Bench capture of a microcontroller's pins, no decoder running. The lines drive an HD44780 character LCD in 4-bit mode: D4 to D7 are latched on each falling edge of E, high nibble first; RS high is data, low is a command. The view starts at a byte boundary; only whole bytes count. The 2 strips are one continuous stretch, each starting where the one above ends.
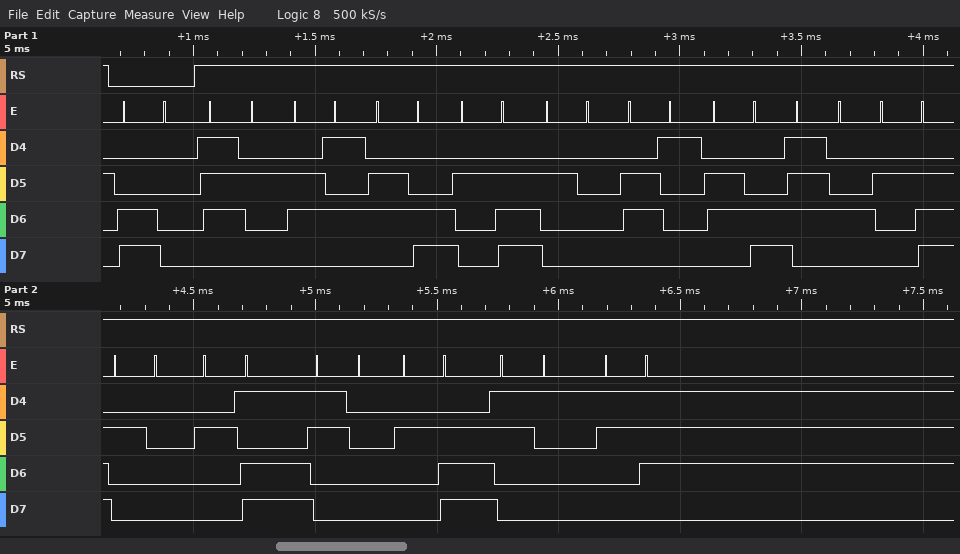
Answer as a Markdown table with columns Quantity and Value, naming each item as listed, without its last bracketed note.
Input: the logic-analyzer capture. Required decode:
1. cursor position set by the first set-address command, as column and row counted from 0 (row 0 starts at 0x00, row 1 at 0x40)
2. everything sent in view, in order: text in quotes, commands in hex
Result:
| Quantity | Value |
|---|---|
| cursor position set by the first set-address command, as column and row counted from 0 | column 0, row 1 |
| everything sent in view, in order: text in quotes, commands in hex | 0xC0 "rel. alt. -0.17" |
